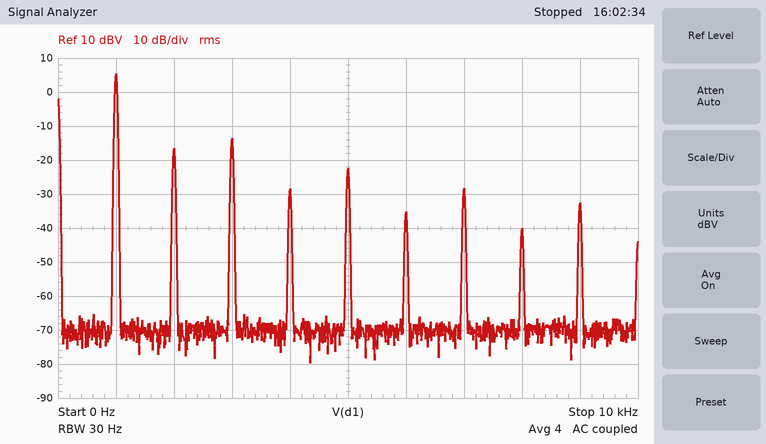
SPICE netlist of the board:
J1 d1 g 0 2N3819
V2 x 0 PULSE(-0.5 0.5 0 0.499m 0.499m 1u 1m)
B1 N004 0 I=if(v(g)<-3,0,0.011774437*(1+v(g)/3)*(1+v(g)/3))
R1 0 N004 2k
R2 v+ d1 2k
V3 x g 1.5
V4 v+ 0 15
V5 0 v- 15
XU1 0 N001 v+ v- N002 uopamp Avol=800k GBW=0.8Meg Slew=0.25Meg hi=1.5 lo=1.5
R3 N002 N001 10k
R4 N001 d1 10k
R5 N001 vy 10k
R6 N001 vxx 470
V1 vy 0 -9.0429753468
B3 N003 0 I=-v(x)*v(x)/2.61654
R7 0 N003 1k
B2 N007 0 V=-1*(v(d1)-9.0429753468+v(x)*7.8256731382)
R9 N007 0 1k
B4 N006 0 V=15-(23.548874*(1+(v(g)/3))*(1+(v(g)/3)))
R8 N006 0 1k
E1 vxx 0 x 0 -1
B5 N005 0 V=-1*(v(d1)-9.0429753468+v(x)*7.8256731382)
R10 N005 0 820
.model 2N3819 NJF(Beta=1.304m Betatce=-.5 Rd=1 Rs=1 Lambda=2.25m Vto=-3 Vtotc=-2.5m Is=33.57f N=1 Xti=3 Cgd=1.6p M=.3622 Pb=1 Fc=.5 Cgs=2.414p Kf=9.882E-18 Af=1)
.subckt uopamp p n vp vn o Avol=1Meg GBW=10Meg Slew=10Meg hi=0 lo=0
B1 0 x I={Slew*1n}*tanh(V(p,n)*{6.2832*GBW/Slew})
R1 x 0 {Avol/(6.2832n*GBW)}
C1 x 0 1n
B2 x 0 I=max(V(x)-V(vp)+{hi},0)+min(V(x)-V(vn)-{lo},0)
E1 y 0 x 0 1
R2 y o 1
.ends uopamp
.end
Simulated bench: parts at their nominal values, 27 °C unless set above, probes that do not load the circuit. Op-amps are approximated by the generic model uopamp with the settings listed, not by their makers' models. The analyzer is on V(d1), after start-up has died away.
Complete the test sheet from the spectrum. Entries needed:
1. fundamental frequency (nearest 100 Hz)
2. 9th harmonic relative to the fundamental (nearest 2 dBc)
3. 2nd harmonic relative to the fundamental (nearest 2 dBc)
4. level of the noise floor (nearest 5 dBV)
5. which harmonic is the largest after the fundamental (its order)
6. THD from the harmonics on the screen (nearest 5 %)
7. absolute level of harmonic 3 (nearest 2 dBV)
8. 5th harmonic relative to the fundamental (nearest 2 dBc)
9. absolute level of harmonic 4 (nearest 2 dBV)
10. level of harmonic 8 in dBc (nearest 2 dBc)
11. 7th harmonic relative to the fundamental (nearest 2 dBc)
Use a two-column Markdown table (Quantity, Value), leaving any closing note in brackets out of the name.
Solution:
| Quantity | Value |
|---|---|
| fundamental frequency | 1.0 kHz |
| 9th harmonic relative to the fundamental | -38 dBc |
| 2nd harmonic relative to the fundamental | -22 dBc |
| level of the noise floor | -70 dBV |
| which harmonic is the largest after the fundamental | 3 |
| THD from the harmonics on the screen | 15 % |
| absolute level of harmonic 3 | -14 dBV |
| 5th harmonic relative to the fundamental | -28 dBc |
| absolute level of harmonic 4 | -28 dBV |
| level of harmonic 8 in dBc | -46 dBc |
| 7th harmonic relative to the fundamental | -34 dBc |
